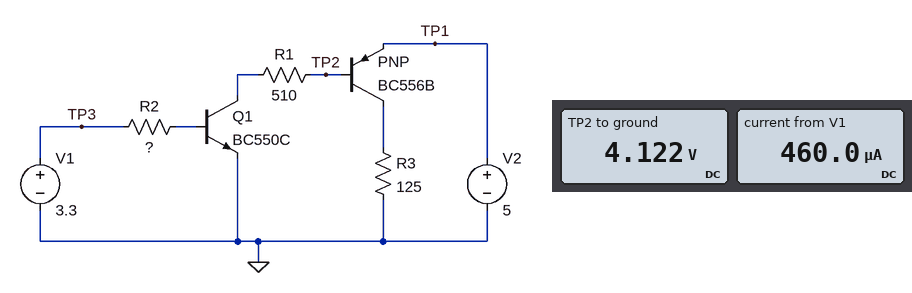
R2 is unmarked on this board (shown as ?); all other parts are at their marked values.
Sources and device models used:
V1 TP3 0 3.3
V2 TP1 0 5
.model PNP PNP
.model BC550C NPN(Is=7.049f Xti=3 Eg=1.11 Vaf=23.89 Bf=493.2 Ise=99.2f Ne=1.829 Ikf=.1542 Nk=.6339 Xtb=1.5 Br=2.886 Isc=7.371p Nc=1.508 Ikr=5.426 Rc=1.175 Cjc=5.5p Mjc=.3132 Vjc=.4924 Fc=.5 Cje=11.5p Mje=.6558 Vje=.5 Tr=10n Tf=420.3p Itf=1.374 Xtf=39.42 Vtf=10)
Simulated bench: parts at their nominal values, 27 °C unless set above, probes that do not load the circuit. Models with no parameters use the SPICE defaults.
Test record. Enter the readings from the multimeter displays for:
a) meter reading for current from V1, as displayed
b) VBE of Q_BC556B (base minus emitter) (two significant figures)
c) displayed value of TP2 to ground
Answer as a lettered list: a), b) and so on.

a) 460.0 µA
b) -880 mV
c) 4.122 V
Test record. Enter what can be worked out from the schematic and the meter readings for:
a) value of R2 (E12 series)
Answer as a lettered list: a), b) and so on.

a) 5.6 kΩ
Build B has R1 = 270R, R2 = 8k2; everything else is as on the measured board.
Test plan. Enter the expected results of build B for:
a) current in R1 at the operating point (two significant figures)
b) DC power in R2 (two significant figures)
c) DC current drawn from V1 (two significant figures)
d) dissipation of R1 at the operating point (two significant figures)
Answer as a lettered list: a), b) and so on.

a) 15 mA
b) 800 µW
c) 310 µA
d) 59 mW
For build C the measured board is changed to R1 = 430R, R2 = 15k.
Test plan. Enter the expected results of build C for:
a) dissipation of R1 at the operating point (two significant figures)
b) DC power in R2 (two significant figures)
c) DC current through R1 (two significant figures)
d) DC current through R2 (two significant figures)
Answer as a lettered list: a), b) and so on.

a) 37 mW
b) 440 µW
c) 9.3 mA
d) 170 µA
